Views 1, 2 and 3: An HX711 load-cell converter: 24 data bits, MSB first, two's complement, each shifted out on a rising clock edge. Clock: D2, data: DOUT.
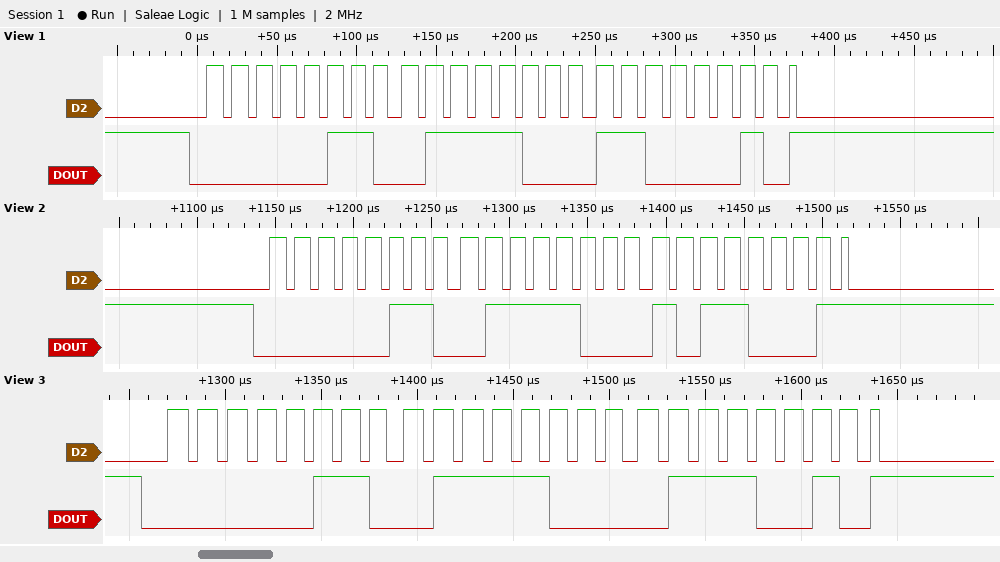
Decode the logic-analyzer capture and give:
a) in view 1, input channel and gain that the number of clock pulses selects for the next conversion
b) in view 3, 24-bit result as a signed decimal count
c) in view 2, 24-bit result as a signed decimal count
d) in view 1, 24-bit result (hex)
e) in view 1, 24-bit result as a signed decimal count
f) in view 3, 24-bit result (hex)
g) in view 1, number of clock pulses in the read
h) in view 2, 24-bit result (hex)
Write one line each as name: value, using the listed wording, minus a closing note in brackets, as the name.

in view 1, input channel and gain that the number of clock pulses selects for the next conversion: channel A, gain 128
in view 3, 24-bit result as a signed decimal count: 424050
in view 2, 24-bit result as a signed decimal count: 424113
in view 1, 24-bit result: 0x0678C2
in view 1, 24-bit result as a signed decimal count: 424130
in view 3, 24-bit result: 0x067872
in view 1, number of clock pulses in the read: 25
in view 2, 24-bit result: 0x0678B1
